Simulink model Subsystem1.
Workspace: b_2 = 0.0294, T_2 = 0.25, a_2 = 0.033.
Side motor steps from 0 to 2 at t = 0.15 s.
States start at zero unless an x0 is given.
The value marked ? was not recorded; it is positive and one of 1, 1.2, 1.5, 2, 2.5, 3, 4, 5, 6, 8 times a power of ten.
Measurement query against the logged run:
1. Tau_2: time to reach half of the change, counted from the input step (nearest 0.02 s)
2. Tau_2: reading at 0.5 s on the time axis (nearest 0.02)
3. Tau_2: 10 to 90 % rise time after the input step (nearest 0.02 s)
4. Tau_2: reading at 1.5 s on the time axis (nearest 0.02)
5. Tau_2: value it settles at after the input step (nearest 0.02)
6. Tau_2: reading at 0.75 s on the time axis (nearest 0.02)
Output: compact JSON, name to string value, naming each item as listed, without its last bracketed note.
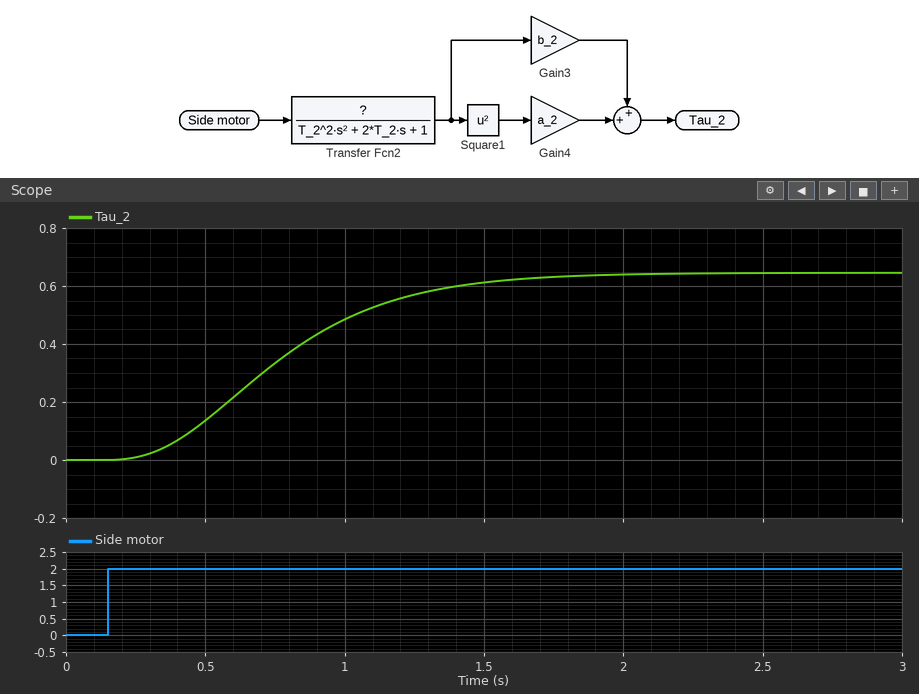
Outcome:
{"Tau_2: time to reach half of the change, counted from the input step": "0.58 s", "Tau_2: reading at 0.5 s on the time axis": "0.14", "Tau_2: 10 to 90 % rise time after the input step": "0.90 s", "Tau_2: reading at 1.5 s on the time axis": "0.62", "Tau_2: value it settles at after the input step": "0.64", "Tau_2: reading at 0.75 s on the time axis": "0.34"}
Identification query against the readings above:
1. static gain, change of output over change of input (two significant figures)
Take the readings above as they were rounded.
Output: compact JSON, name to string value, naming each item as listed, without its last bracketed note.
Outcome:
{"static gain, change of output over change of input": "0.32"}
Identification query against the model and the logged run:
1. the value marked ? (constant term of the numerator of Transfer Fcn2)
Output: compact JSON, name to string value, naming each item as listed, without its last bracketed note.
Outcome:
{"the value marked ?": "2"}
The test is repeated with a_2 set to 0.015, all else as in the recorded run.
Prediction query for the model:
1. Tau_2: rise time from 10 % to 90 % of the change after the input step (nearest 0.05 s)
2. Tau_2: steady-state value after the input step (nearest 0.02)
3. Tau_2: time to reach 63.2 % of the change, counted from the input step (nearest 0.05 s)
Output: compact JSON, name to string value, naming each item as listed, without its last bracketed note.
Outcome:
{"Tau_2: rise time from 10 % to 90 % of the change after the input step": "0.90 s", "Tau_2: steady-state value after the input step": "0.36", "Tau_2: time to reach 63.2 % of the change, counted from the input step": "0.70 s"}
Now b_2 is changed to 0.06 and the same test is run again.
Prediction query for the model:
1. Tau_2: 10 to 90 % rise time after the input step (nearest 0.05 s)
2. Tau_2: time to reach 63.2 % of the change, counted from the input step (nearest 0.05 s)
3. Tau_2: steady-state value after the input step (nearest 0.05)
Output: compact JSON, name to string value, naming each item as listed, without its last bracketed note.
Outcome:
{"Tau_2: 10 to 90 % rise time after the input step": "0.90 s", "Tau_2: time to reach 63.2 % of the change, counted from the input step": "0.70 s", "Tau_2: steady-state value after the input step": "0.75"}
